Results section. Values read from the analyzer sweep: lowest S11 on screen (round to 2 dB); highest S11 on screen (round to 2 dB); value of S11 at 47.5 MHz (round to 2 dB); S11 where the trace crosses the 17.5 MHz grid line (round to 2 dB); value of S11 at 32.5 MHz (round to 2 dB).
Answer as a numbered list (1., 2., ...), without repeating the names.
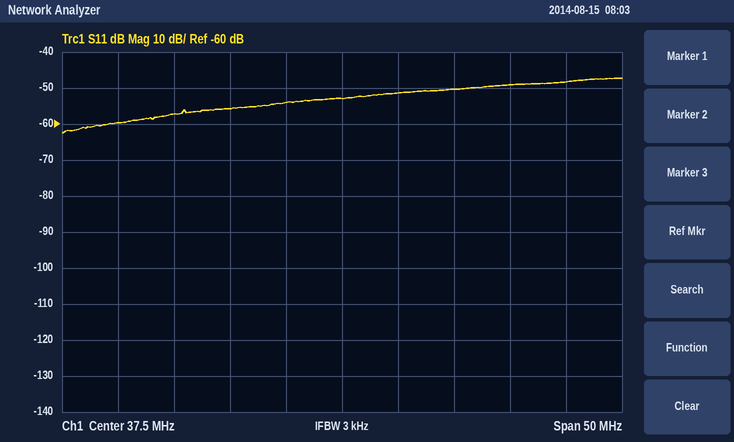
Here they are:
1. -62 dB
2. -48 dB
3. -50 dB
4. -60 dB
5. -54 dB
